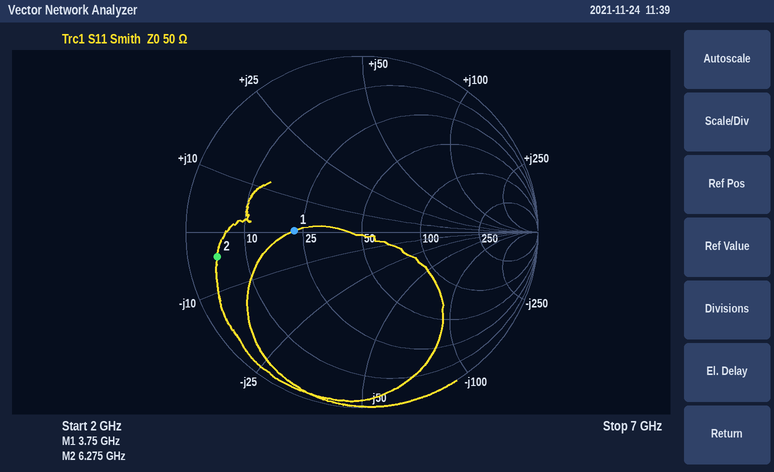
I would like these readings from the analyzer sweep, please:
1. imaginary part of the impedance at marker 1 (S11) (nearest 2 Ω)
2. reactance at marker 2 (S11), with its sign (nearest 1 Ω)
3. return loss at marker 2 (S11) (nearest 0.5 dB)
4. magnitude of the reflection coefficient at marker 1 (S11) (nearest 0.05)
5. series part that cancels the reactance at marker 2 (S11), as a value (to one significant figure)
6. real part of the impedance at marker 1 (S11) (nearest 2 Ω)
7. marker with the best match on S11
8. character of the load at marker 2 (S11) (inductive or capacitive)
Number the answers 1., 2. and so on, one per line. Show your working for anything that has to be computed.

1. 0 Ω
2. -4 Ω
3. 1.5 dB
4. 0.40
5. L = 4 Ω/(2π × 6.275 GHz) ≈ 101 pH, so 100 pH to one significant figure
6. 22 Ω
7. marker 1
8. capacitive
